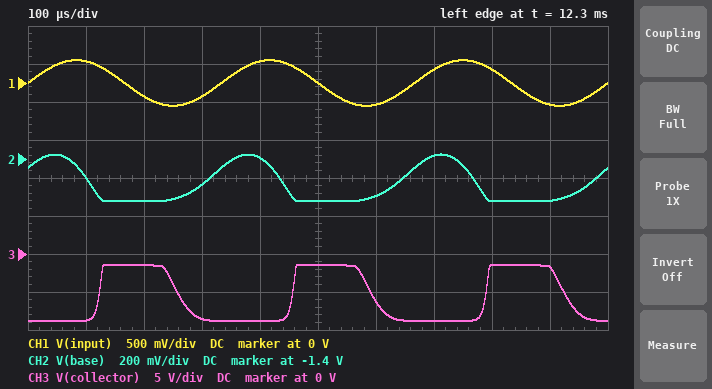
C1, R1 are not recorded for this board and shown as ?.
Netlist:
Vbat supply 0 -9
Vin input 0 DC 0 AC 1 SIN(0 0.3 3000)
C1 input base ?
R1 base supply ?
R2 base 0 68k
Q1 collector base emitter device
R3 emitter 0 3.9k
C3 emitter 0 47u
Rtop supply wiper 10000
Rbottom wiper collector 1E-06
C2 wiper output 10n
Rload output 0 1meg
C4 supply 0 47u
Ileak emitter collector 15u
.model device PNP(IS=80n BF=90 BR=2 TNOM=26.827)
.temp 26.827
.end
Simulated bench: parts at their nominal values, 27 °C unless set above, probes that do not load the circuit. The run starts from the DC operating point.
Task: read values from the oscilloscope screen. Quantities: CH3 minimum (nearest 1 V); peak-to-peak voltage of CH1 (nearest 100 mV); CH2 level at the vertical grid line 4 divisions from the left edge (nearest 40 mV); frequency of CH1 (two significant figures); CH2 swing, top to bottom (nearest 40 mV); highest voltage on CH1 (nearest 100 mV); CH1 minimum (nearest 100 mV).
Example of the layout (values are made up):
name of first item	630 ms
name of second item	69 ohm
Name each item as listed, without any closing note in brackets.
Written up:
CH3 minimum	-9 V
peak-to-peak voltage of CH1	600 mV
CH2 level at the vertical grid line 4 divisions from the left edge	-1.40 V
frequency of CH1	3.0 kHz
CH2 swing, top to bottom	240 mV
highest voltage on CH1	300 mV
CH1 minimum	-300 mV
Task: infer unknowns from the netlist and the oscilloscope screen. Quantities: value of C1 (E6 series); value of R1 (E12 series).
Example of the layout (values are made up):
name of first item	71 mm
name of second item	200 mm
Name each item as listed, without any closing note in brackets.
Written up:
value of C1	2.2 nF
value of R1	270 kΩ
